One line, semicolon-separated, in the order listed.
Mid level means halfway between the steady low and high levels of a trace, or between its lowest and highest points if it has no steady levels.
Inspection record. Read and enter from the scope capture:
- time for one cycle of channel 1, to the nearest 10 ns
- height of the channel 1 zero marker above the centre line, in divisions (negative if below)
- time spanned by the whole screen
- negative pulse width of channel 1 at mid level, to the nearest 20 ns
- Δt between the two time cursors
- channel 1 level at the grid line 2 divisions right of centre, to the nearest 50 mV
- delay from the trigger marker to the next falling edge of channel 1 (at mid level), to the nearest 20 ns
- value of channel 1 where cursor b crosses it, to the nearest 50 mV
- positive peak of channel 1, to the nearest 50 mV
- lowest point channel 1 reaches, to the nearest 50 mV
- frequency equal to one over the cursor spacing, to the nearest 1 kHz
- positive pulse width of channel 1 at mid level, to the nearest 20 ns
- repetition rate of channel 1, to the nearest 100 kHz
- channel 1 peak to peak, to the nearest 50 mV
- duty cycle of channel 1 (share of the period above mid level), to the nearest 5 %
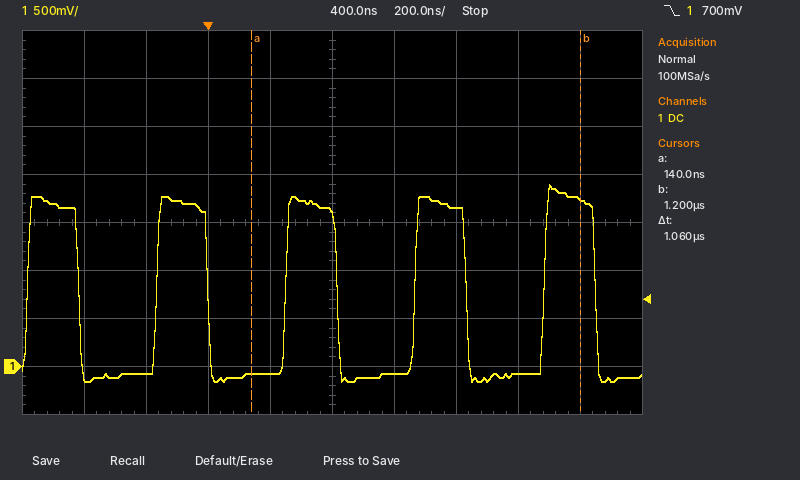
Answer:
420 ns; -3.0 div; 2 µs; 260 ns; 1.06 µs; 1.65 V; 420 ns; 1.75 V; 1.90 V; -150 mV; 943 kHz; 160 ns; 2.4 MHz; 2.05 V; 40 %
